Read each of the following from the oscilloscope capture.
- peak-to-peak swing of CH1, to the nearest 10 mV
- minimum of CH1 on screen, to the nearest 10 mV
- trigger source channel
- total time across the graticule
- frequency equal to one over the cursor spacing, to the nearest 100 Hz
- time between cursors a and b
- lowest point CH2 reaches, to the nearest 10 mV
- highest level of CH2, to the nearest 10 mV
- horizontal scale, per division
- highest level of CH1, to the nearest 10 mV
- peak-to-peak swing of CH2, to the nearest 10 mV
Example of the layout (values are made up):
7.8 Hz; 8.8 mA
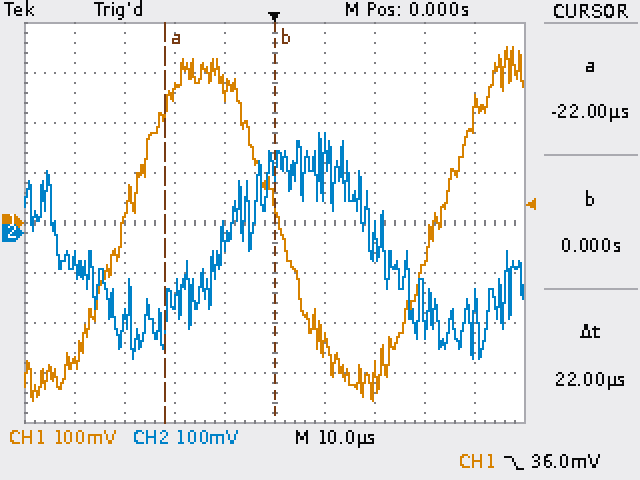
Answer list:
710 mV; -360 mV; CH1; 100 µs; 45.5 kHz; 22 µs; -250 mV; 200 mV; 10 µs; 350 mV; 450 mV
